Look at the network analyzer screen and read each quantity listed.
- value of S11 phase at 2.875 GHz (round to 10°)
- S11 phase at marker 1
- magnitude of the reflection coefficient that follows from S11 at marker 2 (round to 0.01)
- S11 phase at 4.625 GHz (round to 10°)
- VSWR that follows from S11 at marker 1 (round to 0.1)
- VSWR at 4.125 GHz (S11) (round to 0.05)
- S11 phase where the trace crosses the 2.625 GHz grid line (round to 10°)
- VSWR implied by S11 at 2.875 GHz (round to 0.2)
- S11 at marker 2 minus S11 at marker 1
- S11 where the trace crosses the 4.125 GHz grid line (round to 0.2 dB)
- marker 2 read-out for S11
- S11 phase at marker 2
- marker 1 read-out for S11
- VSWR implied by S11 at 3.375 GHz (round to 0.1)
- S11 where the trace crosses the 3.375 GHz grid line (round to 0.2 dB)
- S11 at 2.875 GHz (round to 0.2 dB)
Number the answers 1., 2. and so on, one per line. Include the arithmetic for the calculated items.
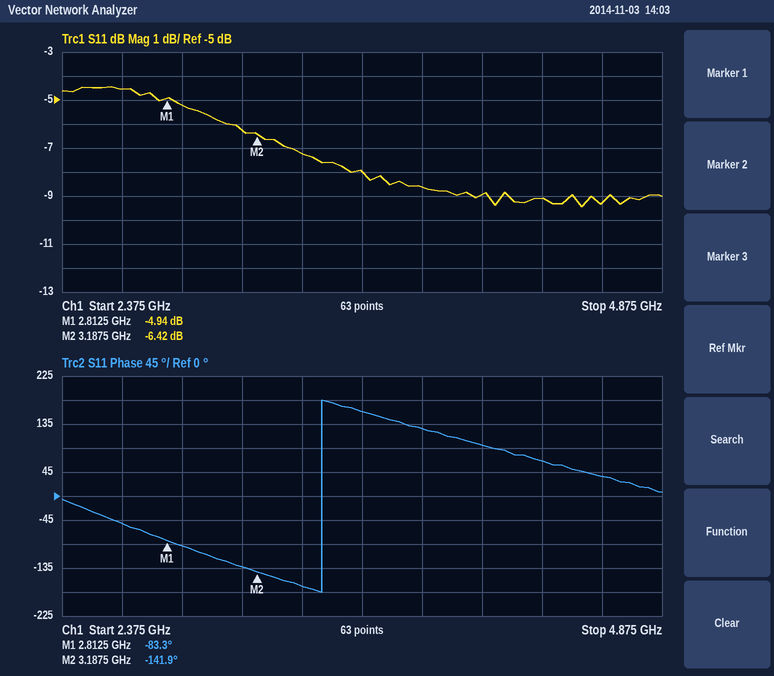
1. -90°
2. -83.3°
3. 10^(-6.42/20) ≈ 0.48
4. 40°
5. (1 + 0.5662)/(1 − 0.5662) ≈ 3.6
6. |Γ| = 10^(-9/20) = 0.3548; VSWR = (1 + 0.3548)/(1 − 0.3548) ≈ 2.10
7. -50°
8. |Γ| = 10^(-5.2/20) = 0.5495; VSWR = (1 + 0.5495)/(1 − 0.5495) ≈ 3.4
9. -6.42 − (-4.94) = -1.48 dB
10. -9.0 dB
11. -6.42 dB
12. -141.9°
13. -4.94 dB
14. |Γ| = 10^(-7.2/20) = 0.4365; VSWR = (1 + 0.4365)/(1 − 0.4365) ≈ 2.5
15. -7.2 dB
16. -5.2 dB
